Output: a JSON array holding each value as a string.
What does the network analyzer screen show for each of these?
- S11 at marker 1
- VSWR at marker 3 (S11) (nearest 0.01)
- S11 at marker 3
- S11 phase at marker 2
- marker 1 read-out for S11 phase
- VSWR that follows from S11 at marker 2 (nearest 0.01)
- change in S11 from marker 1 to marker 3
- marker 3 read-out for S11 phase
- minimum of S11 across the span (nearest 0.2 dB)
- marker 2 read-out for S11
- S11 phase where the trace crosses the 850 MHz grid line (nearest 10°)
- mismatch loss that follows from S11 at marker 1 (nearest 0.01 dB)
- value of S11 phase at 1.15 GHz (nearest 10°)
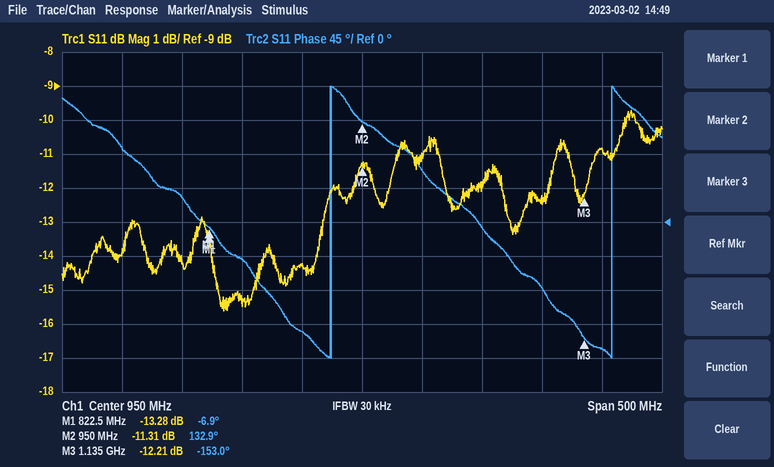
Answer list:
["-13.28 dB", "1.65", "-12.21 dB", "132.9°", "-6.9°", "1.75", "1.07 dB", "-153.0°", "-15.6 dB", "-11.31 dB", "-50°", "0.21 dB", "-170°"]
